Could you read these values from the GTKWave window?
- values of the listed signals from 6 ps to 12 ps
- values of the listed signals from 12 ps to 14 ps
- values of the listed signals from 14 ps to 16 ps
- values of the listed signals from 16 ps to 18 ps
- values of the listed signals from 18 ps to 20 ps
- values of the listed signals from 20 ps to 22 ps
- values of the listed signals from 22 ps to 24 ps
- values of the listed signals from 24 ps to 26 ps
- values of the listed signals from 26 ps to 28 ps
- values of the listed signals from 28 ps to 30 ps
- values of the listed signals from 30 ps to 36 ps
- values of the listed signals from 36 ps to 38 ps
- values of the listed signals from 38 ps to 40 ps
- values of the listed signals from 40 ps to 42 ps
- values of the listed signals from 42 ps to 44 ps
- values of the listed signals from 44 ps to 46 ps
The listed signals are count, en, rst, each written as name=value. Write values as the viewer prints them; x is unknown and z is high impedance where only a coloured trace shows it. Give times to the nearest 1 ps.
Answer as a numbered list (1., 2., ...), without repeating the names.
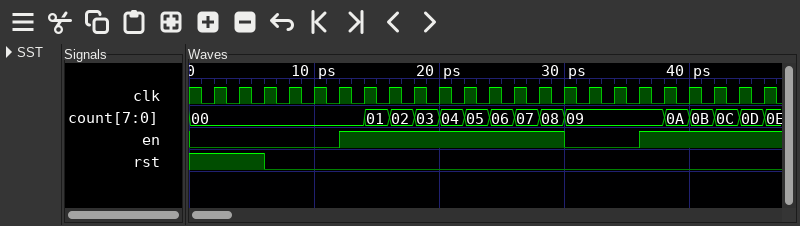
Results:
1. count=00, en=0, rst=0
2. count=00, en=1, rst=0
3. count=01, en=1, rst=0
4. count=02, en=1, rst=0
5. count=03, en=1, rst=0
6. count=04, en=1, rst=0
7. count=05, en=1, rst=0
8. count=06, en=1, rst=0
9. count=07, en=1, rst=0
10. count=08, en=1, rst=0
11. count=09, en=0, rst=0
12. count=09, en=1, rst=0
13. count=0A, en=1, rst=0
14. count=0B, en=1, rst=0
15. count=0C, en=1, rst=0
16. count=0D, en=1, rst=0
